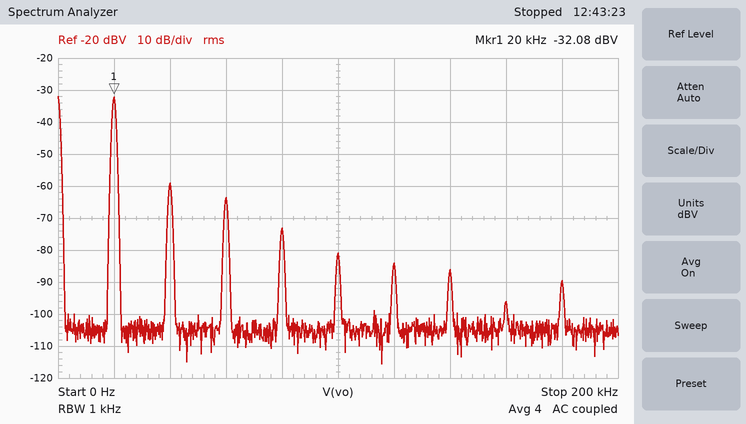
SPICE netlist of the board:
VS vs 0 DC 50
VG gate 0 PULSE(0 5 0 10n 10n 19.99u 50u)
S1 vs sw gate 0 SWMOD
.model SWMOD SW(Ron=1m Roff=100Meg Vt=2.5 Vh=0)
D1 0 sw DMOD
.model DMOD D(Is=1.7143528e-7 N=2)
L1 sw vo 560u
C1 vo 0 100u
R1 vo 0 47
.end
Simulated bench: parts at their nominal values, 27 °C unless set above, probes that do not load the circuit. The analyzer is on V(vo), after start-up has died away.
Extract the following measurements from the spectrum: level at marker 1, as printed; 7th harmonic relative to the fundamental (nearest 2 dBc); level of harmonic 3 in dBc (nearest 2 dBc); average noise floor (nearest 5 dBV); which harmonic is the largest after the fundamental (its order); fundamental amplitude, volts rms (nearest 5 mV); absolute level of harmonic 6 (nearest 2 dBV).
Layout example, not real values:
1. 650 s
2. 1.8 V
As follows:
1. -32.08 dBV
2. -54 dBc
3. -32 dBc
4. -105 dBV
5. 2
6. 25 mV
7. -84 dBV
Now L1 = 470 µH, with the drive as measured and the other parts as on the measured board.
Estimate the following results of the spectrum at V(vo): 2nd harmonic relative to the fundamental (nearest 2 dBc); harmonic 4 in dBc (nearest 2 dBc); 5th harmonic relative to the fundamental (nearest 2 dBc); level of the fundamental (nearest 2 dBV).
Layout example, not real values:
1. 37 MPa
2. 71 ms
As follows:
1. -30 dBc
2. -40 dBc
3. -50 dBc
4. -30 dBV
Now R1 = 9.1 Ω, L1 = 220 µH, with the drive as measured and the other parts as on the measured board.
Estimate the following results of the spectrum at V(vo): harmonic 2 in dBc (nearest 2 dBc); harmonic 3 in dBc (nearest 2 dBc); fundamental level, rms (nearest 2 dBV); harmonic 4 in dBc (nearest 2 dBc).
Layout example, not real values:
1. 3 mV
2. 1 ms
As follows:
1. -22 dBc
2. -32 dBc
3. -24 dBV
4. -36 dBc
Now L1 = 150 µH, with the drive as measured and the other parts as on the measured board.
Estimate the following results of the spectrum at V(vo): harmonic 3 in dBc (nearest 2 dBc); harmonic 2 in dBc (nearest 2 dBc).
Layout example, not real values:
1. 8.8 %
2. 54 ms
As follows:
1. -26 dBc
2. -16 dBc
